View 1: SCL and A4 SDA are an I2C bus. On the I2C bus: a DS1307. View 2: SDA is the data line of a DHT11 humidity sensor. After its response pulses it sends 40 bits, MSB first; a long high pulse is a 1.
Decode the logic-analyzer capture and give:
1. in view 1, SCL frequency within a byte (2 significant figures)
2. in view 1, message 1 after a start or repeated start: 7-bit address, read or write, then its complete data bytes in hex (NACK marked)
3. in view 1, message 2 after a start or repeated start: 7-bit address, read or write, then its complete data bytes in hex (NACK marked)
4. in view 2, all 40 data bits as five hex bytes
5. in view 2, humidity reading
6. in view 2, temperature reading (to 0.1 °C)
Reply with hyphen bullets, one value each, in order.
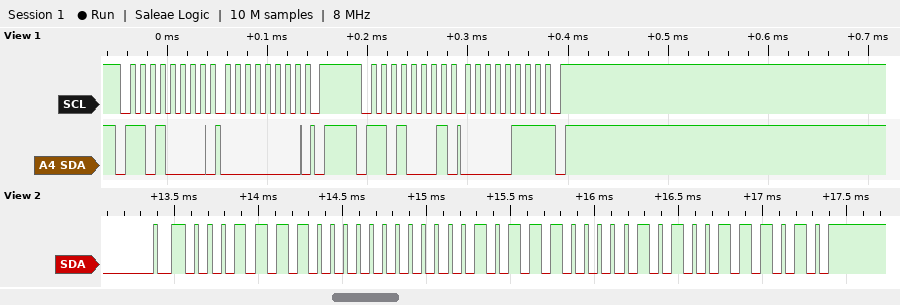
- 100 kHz
- 0x68 write: 00
- 0x68 read: 07 NACK
- 1E 00 17 05 3A
- 30 %
- 23.5 °C
